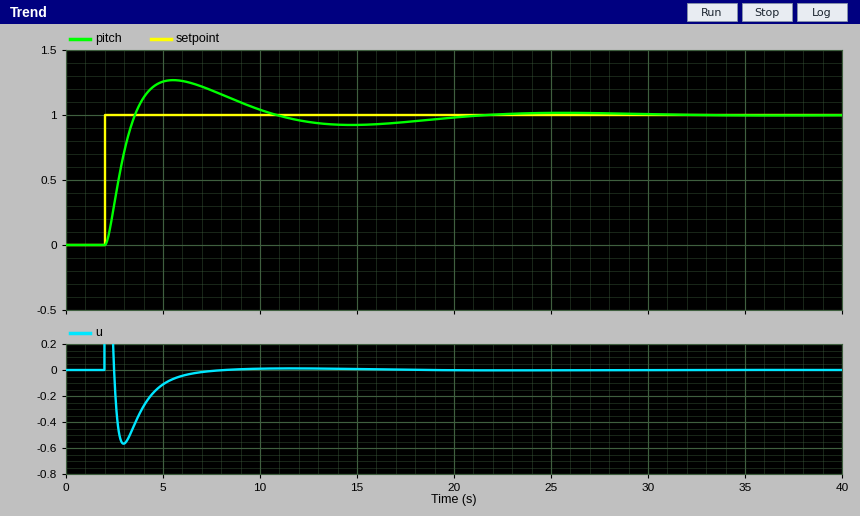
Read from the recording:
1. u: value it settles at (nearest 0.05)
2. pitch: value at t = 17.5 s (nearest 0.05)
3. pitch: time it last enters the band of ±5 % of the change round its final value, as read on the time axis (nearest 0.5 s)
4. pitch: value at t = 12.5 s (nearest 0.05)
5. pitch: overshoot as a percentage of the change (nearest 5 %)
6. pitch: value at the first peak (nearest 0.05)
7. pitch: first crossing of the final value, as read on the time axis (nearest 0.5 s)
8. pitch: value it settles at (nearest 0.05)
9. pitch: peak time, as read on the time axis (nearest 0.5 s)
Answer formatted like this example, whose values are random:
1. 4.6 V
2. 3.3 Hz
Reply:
1. 0.00
2. 0.95
3. 18.0 s
4. 0.95
5. 25 %
6. 1.25
7. 3.5 s
8. 1.00
9. 5.5 s
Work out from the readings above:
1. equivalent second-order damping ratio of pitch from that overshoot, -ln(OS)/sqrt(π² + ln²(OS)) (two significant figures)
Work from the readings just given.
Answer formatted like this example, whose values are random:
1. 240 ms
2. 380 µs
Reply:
1. 0.40
